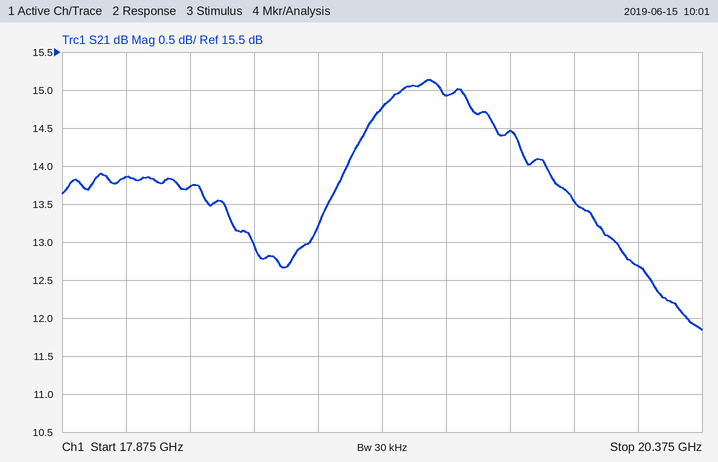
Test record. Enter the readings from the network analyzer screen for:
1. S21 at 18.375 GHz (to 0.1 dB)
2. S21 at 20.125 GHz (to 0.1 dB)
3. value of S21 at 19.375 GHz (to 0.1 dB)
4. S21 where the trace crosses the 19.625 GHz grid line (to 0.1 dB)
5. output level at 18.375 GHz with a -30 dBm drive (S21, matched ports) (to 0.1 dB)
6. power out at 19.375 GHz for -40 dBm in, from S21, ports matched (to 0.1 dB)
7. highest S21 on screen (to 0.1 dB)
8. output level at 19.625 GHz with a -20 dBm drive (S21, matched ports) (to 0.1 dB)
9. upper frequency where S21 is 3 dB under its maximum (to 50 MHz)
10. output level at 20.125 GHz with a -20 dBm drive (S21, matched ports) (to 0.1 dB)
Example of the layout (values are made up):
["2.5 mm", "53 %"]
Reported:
["13.7 dB", "12.7 dB", "14.9 dB", "14.5 dB", "-16.3 dBm", "-25.1 dBm", "15.1 dB", "-5.5 dBm", "20.30 GHz", "-7.3 dBm"]
